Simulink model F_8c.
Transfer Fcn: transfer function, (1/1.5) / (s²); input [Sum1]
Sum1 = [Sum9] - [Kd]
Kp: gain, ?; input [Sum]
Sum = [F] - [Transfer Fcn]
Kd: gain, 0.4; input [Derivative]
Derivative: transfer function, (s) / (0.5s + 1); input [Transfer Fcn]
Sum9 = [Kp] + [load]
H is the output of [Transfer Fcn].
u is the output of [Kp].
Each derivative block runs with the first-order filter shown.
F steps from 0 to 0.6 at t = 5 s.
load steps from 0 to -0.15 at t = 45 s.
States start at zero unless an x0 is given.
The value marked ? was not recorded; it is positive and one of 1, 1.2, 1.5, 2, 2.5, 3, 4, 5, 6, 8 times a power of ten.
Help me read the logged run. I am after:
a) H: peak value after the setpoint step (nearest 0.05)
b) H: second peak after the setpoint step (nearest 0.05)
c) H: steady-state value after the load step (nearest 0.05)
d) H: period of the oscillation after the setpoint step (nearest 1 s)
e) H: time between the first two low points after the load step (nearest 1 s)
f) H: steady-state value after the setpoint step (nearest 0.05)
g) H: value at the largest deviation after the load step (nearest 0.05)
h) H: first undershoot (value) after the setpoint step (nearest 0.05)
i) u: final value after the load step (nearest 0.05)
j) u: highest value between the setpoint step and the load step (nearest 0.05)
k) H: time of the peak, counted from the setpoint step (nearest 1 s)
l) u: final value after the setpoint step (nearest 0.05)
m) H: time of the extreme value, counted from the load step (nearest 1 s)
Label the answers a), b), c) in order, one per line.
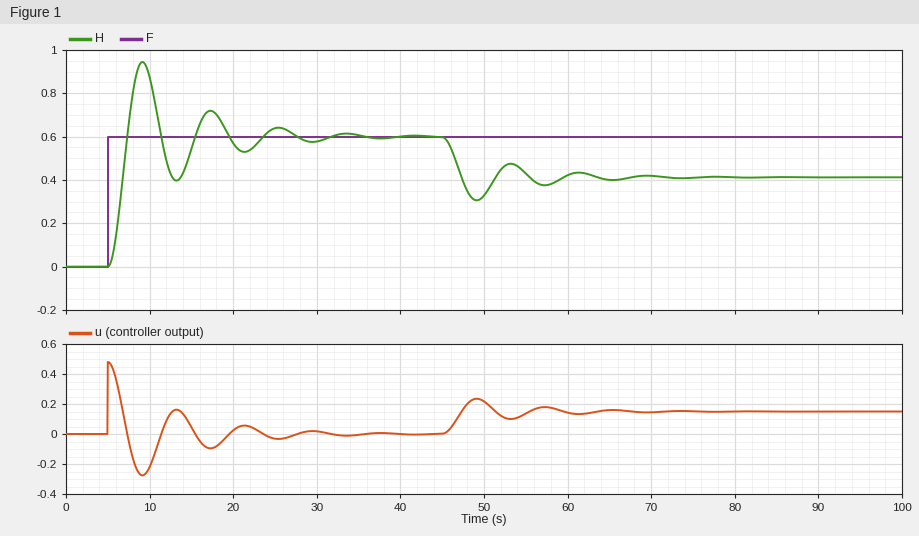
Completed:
a) 0.95
b) 0.70
c) 0.40
d) 8 s
e) 8 s
f) 0.60
g) 0.30
h) 0.40
i) 0.15
j) 0.50
k) 4 s
l) 0.00
m) 4 s
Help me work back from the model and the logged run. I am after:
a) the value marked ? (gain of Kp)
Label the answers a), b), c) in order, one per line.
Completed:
a) 0.8
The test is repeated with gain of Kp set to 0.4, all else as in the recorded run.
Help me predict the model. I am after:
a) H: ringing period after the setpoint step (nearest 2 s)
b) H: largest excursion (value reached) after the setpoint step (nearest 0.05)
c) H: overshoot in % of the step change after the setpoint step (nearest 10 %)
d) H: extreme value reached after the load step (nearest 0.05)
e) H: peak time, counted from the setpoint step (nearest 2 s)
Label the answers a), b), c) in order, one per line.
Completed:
a) 12 s
b) 0.85
c) 40 %
d) 0.05
e) 6 s
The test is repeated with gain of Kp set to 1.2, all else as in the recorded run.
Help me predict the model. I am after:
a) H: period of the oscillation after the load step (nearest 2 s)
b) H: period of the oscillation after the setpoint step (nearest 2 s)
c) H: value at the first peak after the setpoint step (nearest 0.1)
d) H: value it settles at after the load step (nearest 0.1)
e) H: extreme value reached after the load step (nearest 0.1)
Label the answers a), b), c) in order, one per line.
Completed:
a) 6 s
b) 6 s
c) 1.0
d) 0.5
e) 0.4
